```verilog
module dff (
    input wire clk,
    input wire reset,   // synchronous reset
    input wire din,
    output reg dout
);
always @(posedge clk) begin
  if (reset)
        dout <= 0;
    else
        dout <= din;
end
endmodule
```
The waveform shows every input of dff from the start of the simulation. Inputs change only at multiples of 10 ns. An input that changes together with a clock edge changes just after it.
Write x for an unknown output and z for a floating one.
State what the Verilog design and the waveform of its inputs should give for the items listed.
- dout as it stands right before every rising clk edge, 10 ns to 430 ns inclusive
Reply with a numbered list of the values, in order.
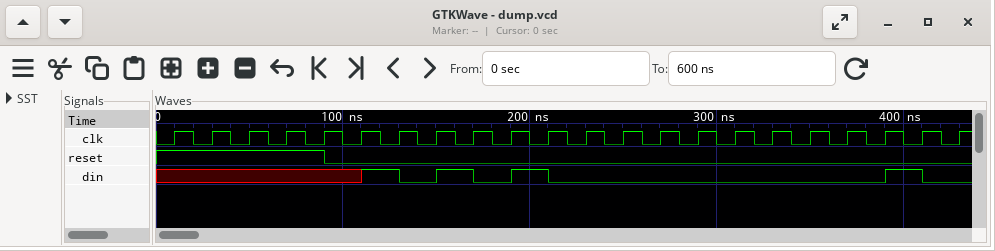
1. x 0 0 0 0 0 x 1 0 1 0 1 0 0 0 0 0 0 0 0 0 1
